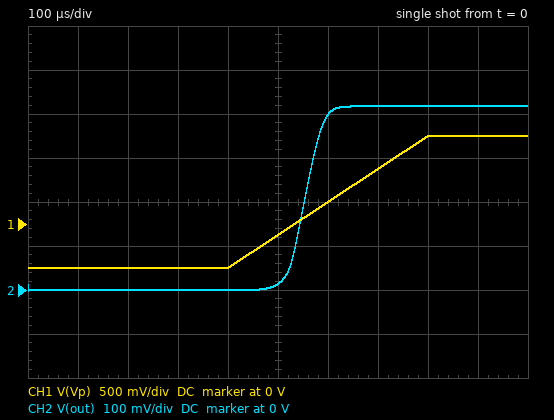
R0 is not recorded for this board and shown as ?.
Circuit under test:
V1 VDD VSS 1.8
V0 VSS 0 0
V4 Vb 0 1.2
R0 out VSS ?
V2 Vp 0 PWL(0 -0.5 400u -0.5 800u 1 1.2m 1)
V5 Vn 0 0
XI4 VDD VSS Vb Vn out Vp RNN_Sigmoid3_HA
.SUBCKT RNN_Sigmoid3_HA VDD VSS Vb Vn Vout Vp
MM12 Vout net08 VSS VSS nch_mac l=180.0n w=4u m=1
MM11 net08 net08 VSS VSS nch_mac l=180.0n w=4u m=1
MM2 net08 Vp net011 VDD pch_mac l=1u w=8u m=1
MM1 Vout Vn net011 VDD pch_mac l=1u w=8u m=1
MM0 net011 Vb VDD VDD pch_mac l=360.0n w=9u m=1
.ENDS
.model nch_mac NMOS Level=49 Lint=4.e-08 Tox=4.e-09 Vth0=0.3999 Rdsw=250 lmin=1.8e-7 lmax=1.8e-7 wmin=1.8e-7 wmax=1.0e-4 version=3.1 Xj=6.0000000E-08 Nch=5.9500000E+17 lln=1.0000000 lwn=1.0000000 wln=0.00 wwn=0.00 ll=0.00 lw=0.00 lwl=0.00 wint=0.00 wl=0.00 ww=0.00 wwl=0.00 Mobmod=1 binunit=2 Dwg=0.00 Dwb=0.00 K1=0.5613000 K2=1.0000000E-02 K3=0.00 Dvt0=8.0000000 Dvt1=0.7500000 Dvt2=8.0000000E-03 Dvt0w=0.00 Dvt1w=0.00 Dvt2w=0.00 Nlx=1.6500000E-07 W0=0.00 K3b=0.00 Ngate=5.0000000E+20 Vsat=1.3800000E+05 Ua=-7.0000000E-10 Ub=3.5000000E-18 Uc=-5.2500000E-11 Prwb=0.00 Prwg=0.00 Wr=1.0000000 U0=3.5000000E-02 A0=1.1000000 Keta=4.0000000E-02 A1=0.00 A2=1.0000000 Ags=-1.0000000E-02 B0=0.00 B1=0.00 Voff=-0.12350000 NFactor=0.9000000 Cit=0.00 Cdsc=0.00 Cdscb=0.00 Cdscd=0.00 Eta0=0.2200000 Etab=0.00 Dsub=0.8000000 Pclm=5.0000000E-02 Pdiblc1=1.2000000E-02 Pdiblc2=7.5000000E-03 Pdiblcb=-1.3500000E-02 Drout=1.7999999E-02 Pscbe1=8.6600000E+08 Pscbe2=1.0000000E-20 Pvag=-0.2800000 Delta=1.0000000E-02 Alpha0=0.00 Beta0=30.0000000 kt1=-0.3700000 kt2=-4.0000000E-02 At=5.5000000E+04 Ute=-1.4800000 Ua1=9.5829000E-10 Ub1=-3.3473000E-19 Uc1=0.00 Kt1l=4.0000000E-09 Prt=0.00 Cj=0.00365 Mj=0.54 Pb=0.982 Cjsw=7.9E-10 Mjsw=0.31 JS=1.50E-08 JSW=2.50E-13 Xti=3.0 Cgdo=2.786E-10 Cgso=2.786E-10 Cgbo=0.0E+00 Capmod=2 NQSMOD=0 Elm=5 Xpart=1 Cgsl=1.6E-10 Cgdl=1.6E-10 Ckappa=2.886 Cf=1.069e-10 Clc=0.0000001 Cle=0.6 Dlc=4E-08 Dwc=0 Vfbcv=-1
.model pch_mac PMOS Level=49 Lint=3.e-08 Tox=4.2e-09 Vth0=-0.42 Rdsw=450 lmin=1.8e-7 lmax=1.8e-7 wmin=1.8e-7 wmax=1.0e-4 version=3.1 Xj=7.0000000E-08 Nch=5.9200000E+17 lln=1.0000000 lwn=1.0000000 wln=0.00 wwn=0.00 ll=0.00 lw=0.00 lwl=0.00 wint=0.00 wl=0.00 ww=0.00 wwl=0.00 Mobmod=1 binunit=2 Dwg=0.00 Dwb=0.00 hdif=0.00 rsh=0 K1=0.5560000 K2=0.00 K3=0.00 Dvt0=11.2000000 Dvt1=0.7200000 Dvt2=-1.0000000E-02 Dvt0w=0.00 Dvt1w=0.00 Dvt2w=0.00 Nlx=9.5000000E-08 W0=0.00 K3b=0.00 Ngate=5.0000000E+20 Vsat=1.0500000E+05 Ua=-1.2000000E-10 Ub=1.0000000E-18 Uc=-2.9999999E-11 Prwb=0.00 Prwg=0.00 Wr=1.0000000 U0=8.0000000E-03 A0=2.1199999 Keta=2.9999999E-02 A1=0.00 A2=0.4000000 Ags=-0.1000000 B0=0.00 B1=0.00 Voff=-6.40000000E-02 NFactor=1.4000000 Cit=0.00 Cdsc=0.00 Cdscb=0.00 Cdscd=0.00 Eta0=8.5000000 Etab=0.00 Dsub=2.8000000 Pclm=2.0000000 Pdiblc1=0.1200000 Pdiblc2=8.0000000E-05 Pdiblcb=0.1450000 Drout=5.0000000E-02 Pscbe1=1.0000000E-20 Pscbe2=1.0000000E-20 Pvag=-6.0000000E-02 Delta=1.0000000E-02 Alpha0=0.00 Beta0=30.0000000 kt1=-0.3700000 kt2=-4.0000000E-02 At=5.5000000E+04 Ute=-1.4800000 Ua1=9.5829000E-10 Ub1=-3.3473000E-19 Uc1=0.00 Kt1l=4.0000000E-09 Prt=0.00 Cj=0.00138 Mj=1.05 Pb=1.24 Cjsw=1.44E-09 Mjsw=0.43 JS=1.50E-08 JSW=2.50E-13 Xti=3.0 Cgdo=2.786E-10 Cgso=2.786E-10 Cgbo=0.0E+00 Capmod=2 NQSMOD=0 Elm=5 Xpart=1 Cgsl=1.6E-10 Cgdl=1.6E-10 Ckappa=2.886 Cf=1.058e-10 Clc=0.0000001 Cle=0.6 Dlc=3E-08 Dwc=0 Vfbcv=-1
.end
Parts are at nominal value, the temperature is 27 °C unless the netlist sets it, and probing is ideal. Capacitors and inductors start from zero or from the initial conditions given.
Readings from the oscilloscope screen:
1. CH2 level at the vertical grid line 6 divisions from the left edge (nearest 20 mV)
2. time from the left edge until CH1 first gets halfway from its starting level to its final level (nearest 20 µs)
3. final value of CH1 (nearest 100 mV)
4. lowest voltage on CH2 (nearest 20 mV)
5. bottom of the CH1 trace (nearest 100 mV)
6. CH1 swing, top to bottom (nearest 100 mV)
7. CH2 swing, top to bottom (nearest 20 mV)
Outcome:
400 mV
600 µs
1.0 V
0 V
-500 mV
1.5 V
420 mV
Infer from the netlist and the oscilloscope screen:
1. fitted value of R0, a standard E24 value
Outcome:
33 kΩ
